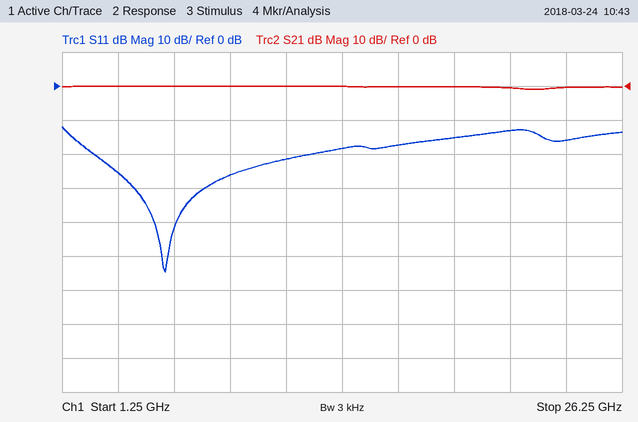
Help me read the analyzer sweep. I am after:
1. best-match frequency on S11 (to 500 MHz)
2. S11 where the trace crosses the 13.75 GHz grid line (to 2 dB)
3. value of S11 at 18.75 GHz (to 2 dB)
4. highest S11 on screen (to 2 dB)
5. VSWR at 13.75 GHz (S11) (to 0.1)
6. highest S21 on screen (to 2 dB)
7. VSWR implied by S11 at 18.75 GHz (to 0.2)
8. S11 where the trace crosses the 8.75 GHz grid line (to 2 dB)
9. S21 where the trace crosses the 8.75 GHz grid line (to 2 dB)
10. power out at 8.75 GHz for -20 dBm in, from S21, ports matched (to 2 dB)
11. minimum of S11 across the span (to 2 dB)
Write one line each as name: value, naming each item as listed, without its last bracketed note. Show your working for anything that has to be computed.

best-match frequency on S11: 6.0 GHz
S11 where the trace crosses the 13.75 GHz grid line: -18 dB
value of S11 at 18.75 GHz: -16 dB
highest S11 on screen: -12 dB
VSWR at 13.75 GHz (S11): |Γ| = 10^(-18/20) = 0.1259; VSWR = (1 + 0.1259)/(1 − 0.1259) ≈ 1.3
highest S21 on screen: 0 dB
VSWR implied by S11 at 18.75 GHz: |Γ| = 10^(-16/20) = 0.1585; VSWR = (1 + 0.1585)/(1 − 0.1585) ≈ 1.4
S11 where the trace crosses the 8.75 GHz grid line: -26 dB
S21 where the trace crosses the 8.75 GHz grid line: 0 dB
power out at 8.75 GHz for -20 dBm in, from S21, ports matched: -20 dBm + (0 dB) = -20 dBm
minimum of S11 across the span: -54 dB
